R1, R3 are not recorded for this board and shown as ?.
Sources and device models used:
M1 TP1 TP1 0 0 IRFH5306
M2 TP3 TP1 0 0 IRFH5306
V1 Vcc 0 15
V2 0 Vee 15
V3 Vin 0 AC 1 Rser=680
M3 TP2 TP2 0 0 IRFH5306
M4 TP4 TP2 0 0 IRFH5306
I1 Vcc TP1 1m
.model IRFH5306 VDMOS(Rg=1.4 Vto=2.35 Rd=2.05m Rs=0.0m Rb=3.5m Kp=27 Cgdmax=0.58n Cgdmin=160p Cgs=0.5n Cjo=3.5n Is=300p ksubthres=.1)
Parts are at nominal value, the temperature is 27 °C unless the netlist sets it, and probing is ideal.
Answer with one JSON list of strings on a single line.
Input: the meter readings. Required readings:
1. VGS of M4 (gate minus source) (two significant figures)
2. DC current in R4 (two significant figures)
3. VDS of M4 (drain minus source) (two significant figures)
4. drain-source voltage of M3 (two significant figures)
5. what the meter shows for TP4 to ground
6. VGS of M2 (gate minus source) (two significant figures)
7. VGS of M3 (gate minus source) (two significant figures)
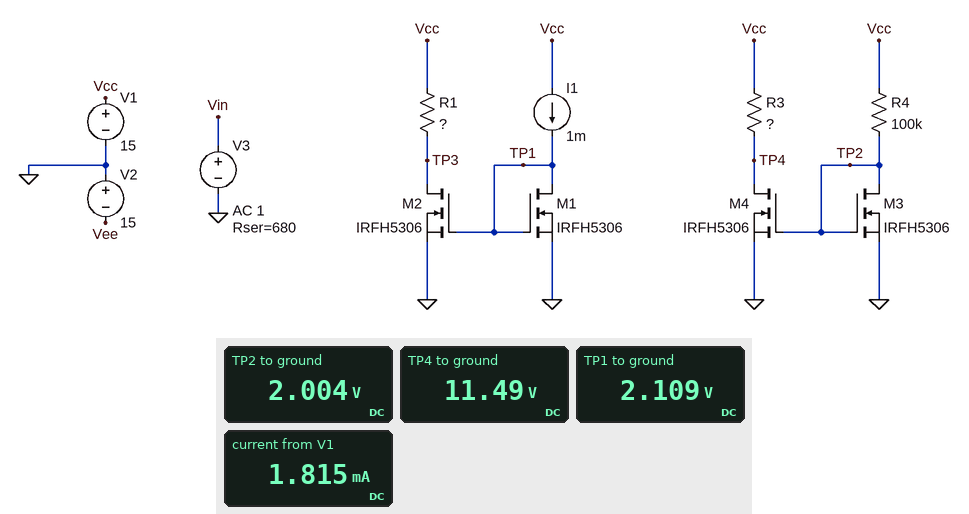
["2.0 V", "130 µA", "11 V", "2.0 V", "11.49 V", "2.1 V", "2.0 V"]
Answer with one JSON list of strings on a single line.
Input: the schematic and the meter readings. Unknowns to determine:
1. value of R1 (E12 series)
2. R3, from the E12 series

["27 kΩ", "27 kΩ"]
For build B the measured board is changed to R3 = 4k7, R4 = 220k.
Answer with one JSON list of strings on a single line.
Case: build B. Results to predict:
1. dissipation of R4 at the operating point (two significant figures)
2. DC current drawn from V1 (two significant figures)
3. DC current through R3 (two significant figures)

["770 µW", "1.7 mA", "59 µA"]
